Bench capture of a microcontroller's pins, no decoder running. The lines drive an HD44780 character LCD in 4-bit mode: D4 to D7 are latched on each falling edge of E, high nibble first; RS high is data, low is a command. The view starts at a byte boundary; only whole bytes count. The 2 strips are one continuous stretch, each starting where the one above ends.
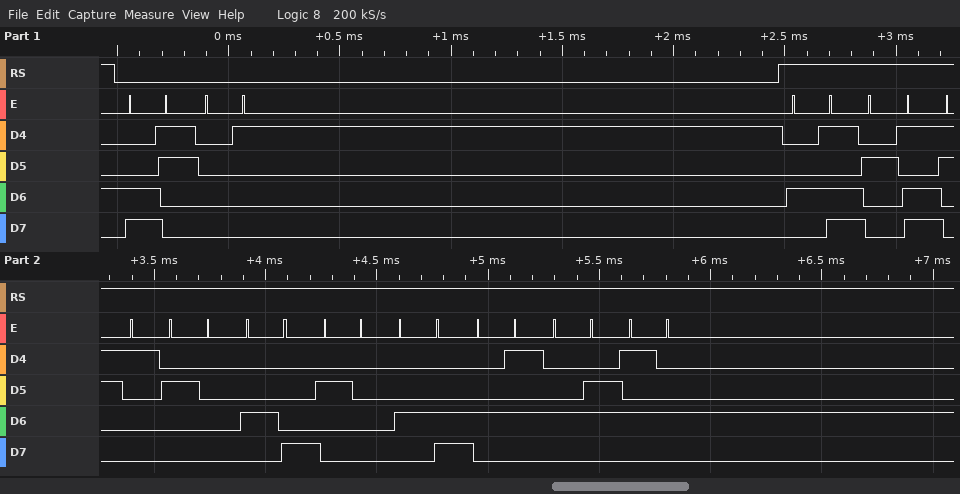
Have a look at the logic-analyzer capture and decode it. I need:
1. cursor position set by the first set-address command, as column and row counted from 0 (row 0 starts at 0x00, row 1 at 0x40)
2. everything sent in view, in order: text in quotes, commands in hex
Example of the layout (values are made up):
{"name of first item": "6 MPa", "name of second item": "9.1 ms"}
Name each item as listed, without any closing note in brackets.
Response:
{"cursor position set by the first set-address command, as column and row counted from 0": "column 3, row 1", "everything sent in view, in order: text in quotes, commands in hex": "0xC3 0x01 \"M-1 H LEFT\""}
